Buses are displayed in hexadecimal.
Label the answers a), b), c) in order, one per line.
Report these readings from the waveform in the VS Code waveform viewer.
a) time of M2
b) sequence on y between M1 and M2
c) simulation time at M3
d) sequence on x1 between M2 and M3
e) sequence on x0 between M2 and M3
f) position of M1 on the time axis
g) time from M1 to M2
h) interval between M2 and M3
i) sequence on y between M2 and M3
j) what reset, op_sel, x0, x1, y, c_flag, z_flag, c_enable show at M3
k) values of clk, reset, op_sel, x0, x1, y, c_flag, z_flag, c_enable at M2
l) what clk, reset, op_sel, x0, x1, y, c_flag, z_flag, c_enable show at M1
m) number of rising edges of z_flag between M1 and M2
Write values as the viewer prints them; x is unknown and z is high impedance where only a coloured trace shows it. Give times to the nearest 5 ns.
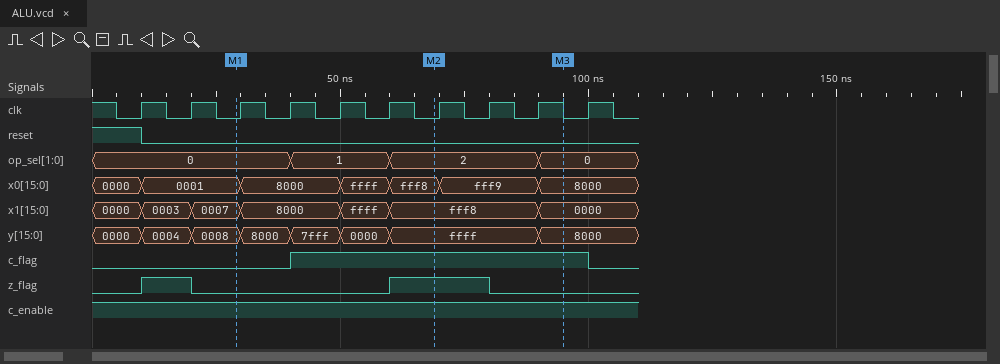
a) 70 ns
b) 0008, 8000, 7fff, 0000, ffff
c) 95 ns
d) fff8, 0000
e) fff8, fff9, 8000
f) 30 ns
g) 40 ns
h) 25 ns
i) ffff, 8000
j) reset=0, op_sel=0, x0=8000, x1=0000, y=8000, c_flag=1, z_flag=0, c_enable=1
k) clk=0, reset=0, op_sel=2, x0=fff8, x1=fff8, y=ffff, c_flag=1, z_flag=1, c_enable=1
l) clk=0, reset=0, op_sel=0, x0=0001, x1=0007, y=0008, c_flag=0, z_flag=0, c_enable=1
m) 1
